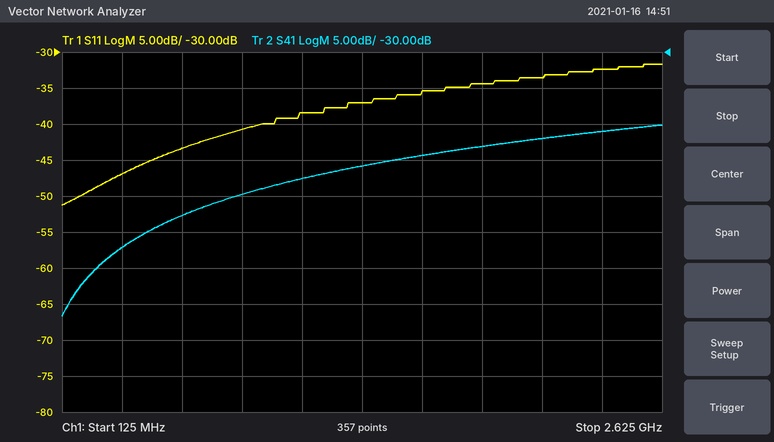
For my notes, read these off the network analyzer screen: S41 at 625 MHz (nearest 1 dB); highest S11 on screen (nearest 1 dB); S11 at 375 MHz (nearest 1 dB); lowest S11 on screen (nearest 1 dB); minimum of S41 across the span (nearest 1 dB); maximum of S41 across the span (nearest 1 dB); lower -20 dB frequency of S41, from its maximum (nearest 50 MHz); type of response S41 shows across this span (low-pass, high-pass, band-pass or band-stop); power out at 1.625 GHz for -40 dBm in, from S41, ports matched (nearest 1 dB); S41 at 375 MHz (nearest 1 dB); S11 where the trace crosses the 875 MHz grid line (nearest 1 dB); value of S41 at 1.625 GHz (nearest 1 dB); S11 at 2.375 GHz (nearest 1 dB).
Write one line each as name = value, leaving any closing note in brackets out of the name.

S41 at 625 MHz = -53 dB
highest S11 on screen = -32 dB
S11 at 375 MHz = -47 dB
lowest S11 on screen = -51 dB
minimum of S41 across the span = -67 dB
maximum of S41 across the span = -40 dB
lower -20 dB frequency of S41, from its maximum = 250 MHz
type of response S41 shows across this span = high-pass
power out at 1.625 GHz for -40 dBm in, from S41, ports matched = -84 dBm
S41 at 375 MHz = -57 dB
S11 where the trace crosses the 875 MHz grid line = -41 dB
value of S41 at 1.625 GHz = -44 dB
S11 at 2.375 GHz = -32 dB
